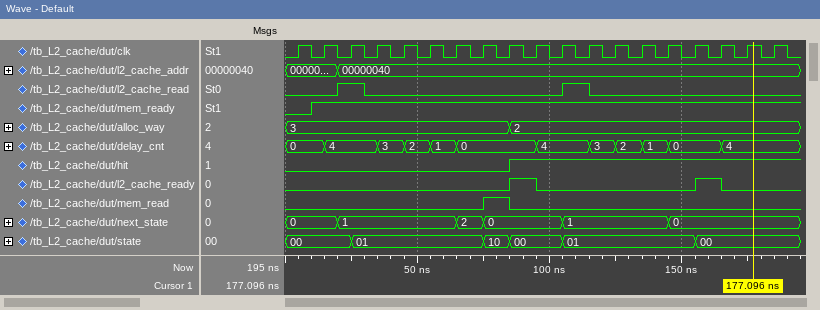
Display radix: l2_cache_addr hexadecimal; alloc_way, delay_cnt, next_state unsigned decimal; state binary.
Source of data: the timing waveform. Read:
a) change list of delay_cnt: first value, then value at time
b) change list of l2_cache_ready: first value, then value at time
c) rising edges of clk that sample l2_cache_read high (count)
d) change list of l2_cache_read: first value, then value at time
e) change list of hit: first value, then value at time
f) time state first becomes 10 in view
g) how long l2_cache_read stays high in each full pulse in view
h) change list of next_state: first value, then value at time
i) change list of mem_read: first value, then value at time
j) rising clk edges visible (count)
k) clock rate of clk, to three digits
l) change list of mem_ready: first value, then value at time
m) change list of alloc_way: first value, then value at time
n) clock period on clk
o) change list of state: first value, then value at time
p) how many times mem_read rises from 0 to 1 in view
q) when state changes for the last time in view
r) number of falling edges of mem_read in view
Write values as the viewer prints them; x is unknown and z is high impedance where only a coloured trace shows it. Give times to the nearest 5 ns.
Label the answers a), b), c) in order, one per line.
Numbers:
a) 0, 4 at 15 ns, 3 at 35 ns, 2 at 45 ns, 1 at 55 ns, 0 at 65 ns, 4 at 95 ns, 3 at 115 ns, 2 at 125 ns, 1 at 135 ns, 0 at 145 ns, 4 at 165 ns
b) 0, 1 at 85 ns, 0 at 95 ns, 1 at 155 ns, 0 at 165 ns
c) 2
d) 0, 1 at 20 ns, 0 at 30 ns, 1 at 105 ns, 0 at 115 ns
e) 0, 1 at 85 ns
f) 75 ns
g) 10 ns, 10 ns
h) 0, 1 at 20 ns, 2 at 65 ns, 0 at 75 ns, 1 at 105 ns, 0 at 145 ns
i) 0, 1 at 75 ns, 0 at 85 ns
j) 19
k) 100 MHz
l) 0, 1 at 10 ns
m) 3, 2 at 85 ns
n) 10 ns
o) 00, 01 at 25 ns, 10 at 75 ns, 00 at 85 ns, 01 at 105 ns, 00 at 155 ns
p) 1
q) 155 ns
r) 1
